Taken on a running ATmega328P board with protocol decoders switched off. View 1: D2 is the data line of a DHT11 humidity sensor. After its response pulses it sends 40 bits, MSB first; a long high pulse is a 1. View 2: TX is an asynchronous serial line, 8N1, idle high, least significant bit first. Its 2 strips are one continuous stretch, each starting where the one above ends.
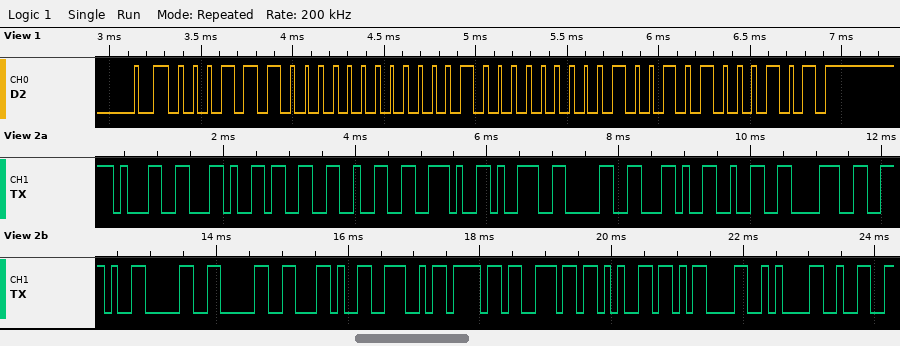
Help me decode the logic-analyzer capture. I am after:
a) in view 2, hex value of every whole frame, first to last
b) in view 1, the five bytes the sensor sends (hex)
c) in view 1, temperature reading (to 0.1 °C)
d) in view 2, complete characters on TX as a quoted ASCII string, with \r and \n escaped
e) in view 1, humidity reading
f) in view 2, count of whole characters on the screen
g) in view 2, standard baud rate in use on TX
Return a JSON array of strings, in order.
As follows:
["31 2C 33 32 2E 39 30 2C 32 38 2E 30 30 2C 4E 6F 6E 65 0D 0A 32", "1C 00 20 09 45", "32.9 °C", "\"1,32.90,28.00,None\\r\\n2\"", "28 %", "21", "9600 baud"]
